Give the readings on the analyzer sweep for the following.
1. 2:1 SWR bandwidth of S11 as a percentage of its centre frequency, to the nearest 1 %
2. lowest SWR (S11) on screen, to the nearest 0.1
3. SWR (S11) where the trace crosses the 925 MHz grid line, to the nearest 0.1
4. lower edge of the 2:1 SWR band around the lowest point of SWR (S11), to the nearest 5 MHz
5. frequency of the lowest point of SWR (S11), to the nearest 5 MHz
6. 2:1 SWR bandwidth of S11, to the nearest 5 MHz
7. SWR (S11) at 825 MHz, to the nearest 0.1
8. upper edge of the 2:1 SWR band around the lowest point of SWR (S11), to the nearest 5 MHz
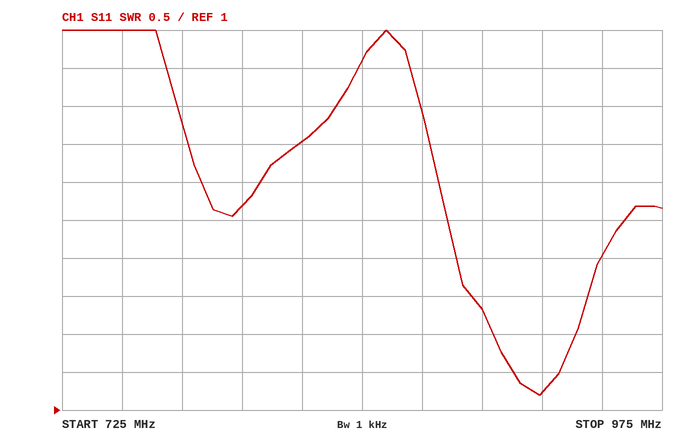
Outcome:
4 %
1.2
1.2
905 MHz
925 MHz
35 MHz
4.5
940 MHz
